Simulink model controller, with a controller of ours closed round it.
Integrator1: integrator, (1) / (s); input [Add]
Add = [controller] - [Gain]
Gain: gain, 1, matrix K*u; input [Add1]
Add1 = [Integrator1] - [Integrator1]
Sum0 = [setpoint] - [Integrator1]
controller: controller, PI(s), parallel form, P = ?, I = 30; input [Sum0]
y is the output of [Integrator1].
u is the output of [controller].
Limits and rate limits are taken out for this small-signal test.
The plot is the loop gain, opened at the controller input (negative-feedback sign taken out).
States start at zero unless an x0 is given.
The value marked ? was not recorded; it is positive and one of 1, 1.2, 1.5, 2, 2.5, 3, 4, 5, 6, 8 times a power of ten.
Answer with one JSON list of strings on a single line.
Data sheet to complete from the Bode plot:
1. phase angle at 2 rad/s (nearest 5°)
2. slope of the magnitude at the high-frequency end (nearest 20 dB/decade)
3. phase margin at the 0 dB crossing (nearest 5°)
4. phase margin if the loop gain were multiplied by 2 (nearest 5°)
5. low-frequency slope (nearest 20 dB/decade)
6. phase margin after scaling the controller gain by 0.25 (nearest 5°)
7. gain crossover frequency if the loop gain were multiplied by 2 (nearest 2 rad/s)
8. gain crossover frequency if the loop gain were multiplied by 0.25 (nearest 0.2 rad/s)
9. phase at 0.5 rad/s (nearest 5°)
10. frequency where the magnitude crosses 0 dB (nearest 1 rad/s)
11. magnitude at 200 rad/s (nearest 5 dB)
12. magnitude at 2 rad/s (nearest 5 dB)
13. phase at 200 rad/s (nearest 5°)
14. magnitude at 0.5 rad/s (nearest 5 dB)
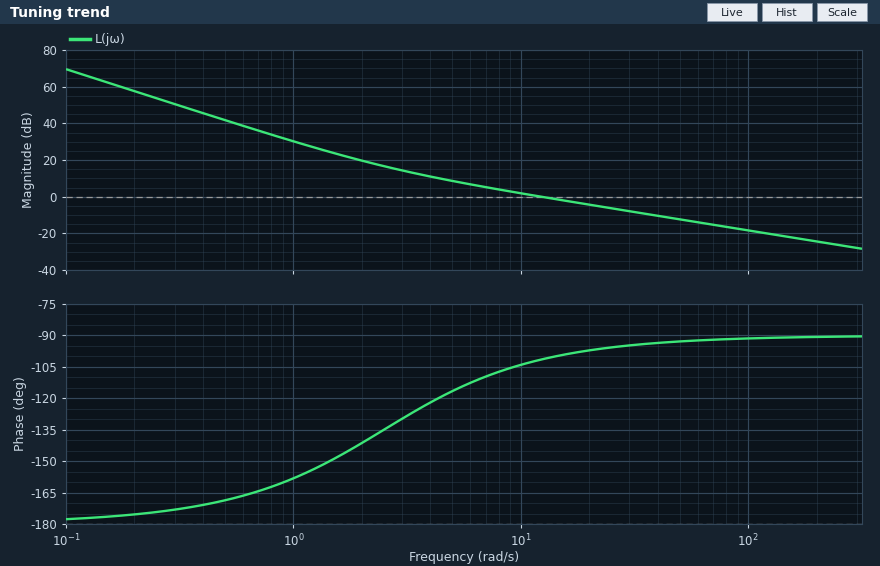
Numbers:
["-140°", "-20 dB/decade", "80°", "85°", "-40 dB/decade", "55°", "24 rad/s", "3.6 rad/s", "-170°", "12 rad/s", "-25 dB", "20 dB", "-90°", "40 dB"]
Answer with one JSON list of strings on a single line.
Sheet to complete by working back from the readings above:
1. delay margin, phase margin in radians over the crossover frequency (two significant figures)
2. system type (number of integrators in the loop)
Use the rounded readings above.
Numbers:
["0.12 s", "2"]
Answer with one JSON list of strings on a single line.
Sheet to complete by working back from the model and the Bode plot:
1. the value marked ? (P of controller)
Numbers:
["12"]
